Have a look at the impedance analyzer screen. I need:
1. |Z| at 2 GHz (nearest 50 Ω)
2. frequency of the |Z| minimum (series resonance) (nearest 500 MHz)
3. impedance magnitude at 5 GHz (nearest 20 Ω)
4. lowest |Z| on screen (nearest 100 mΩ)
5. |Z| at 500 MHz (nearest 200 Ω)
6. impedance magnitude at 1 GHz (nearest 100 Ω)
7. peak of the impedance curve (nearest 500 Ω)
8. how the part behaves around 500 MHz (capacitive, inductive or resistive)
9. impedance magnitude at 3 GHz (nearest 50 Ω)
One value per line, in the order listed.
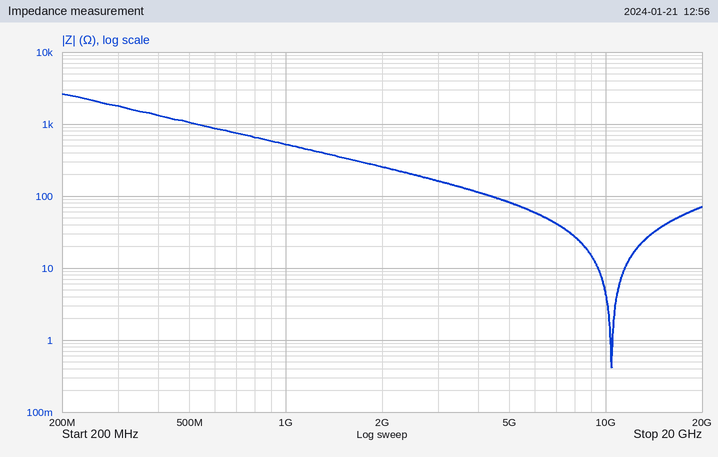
250 Ω
10.5 GHz
80 Ω
400 mΩ
1.0 kΩ
500 Ω
2.5 kΩ
capacitive
150 Ω
